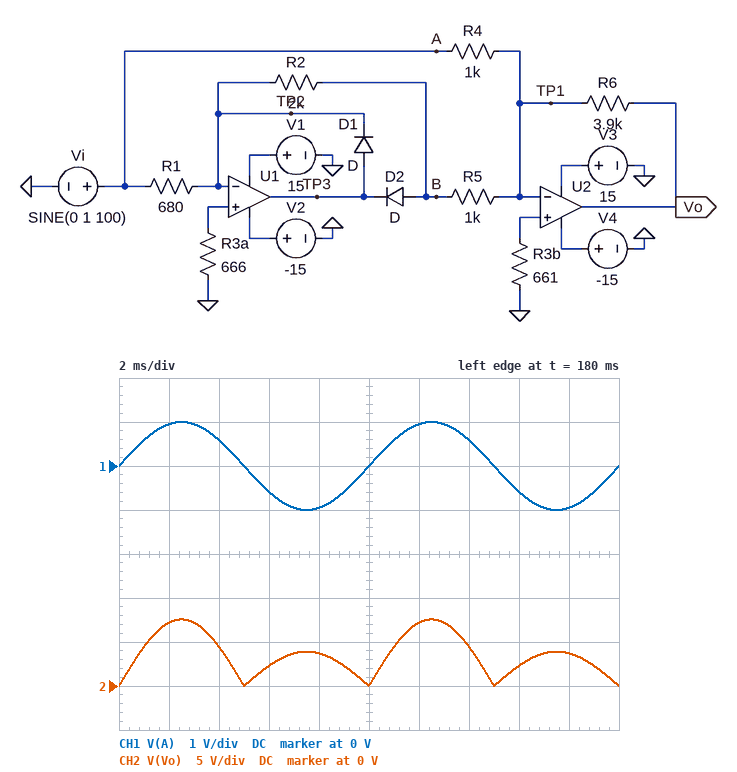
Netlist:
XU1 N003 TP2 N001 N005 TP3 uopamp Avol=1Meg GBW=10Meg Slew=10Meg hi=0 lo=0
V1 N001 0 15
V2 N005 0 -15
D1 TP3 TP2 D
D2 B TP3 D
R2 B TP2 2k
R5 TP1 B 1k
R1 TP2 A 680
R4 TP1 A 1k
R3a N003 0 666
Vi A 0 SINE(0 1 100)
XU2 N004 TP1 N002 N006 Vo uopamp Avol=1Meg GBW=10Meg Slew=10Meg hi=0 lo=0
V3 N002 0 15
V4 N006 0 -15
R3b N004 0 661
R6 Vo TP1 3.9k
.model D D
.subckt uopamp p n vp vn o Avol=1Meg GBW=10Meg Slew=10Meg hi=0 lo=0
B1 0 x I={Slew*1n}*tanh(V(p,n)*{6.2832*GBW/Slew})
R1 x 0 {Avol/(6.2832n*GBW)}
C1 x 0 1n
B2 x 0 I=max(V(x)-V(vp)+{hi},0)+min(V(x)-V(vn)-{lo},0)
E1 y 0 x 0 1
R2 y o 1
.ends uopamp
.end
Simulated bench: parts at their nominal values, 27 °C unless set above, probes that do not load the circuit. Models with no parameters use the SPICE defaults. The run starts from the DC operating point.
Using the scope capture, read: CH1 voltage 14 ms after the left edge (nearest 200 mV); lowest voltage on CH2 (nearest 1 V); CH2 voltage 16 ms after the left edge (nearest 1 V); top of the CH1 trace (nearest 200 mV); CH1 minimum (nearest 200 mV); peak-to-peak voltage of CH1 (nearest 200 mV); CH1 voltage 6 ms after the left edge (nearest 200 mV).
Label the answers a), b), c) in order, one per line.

a) 600 mV
b) 0 V
c) 2 V
d) 1.0 V
e) -1.0 V
f) 2.0 V
g) -600 mV
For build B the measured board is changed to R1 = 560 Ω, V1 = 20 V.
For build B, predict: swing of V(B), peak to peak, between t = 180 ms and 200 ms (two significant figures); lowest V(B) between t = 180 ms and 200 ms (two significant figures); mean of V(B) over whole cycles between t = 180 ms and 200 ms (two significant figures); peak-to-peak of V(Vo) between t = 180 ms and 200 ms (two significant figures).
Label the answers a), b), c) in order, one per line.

a) 3.6 V
b) -3.6 V
c) -1.1 V
d) 10 V
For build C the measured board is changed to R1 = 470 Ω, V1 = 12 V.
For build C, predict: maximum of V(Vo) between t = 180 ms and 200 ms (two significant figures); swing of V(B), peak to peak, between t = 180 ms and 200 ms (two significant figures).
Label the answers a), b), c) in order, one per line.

a) 13 V
b) 4.3 V
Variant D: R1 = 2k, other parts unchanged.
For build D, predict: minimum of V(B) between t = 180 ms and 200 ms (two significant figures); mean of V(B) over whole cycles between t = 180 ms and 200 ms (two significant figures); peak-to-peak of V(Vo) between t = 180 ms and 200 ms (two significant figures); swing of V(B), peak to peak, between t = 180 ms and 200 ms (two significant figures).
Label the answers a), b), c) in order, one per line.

a) -1.0 V
b) -320 mV
c) 3.9 V
d) 1.0 V
